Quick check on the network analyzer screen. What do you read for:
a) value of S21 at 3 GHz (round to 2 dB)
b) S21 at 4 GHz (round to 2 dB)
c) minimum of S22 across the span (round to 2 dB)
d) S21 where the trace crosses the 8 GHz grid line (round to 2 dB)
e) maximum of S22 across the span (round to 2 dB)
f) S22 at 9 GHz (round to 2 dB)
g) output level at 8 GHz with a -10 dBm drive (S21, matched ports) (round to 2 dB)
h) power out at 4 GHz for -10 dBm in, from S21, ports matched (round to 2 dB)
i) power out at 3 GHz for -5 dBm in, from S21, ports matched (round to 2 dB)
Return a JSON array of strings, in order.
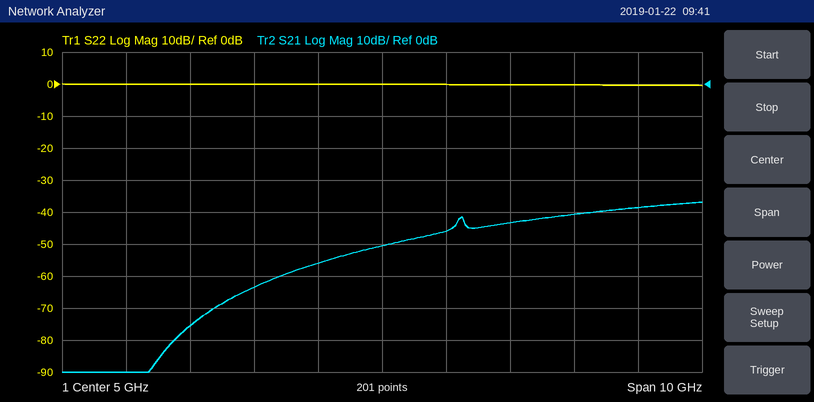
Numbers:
["-64 dB", "-56 dB", "0 dB", "-40 dB", "0 dB", "0 dB", "-50 dBm", "-66 dBm", "-68 dBm"]
